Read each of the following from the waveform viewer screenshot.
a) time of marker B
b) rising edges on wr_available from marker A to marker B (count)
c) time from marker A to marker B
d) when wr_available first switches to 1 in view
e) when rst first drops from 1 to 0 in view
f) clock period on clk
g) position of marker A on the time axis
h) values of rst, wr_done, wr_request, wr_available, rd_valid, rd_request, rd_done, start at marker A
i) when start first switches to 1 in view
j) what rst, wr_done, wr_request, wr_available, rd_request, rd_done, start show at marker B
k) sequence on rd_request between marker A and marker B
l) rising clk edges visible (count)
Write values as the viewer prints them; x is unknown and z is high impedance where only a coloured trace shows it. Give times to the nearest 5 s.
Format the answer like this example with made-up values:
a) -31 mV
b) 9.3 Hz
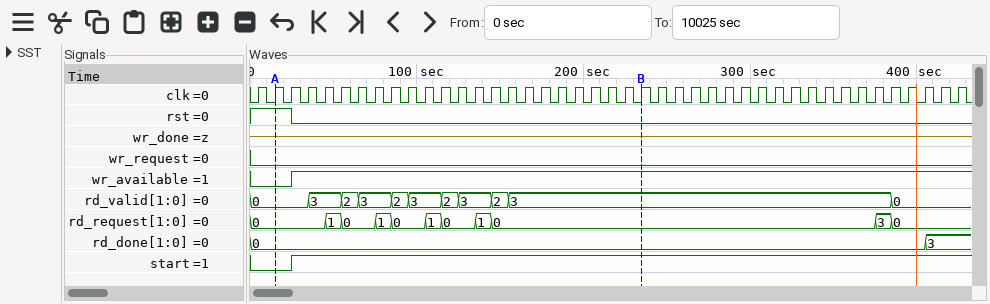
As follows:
a) 235 s
b) 1
c) 220 s
d) 25 s
e) 25 s
f) 10 s
g) 15 s
h) rst=1, wr_done=z, wr_request=0, wr_available=0, rd_valid=0, rd_request=0, rd_done=0, start=0
i) 25 s
j) rst=0, wr_done=z, wr_request=0, wr_available=1, rd_request=0, rd_done=0, start=1
k) 0, 1, 0, 1, 0, 1, 0, 1, 0
l) 43
